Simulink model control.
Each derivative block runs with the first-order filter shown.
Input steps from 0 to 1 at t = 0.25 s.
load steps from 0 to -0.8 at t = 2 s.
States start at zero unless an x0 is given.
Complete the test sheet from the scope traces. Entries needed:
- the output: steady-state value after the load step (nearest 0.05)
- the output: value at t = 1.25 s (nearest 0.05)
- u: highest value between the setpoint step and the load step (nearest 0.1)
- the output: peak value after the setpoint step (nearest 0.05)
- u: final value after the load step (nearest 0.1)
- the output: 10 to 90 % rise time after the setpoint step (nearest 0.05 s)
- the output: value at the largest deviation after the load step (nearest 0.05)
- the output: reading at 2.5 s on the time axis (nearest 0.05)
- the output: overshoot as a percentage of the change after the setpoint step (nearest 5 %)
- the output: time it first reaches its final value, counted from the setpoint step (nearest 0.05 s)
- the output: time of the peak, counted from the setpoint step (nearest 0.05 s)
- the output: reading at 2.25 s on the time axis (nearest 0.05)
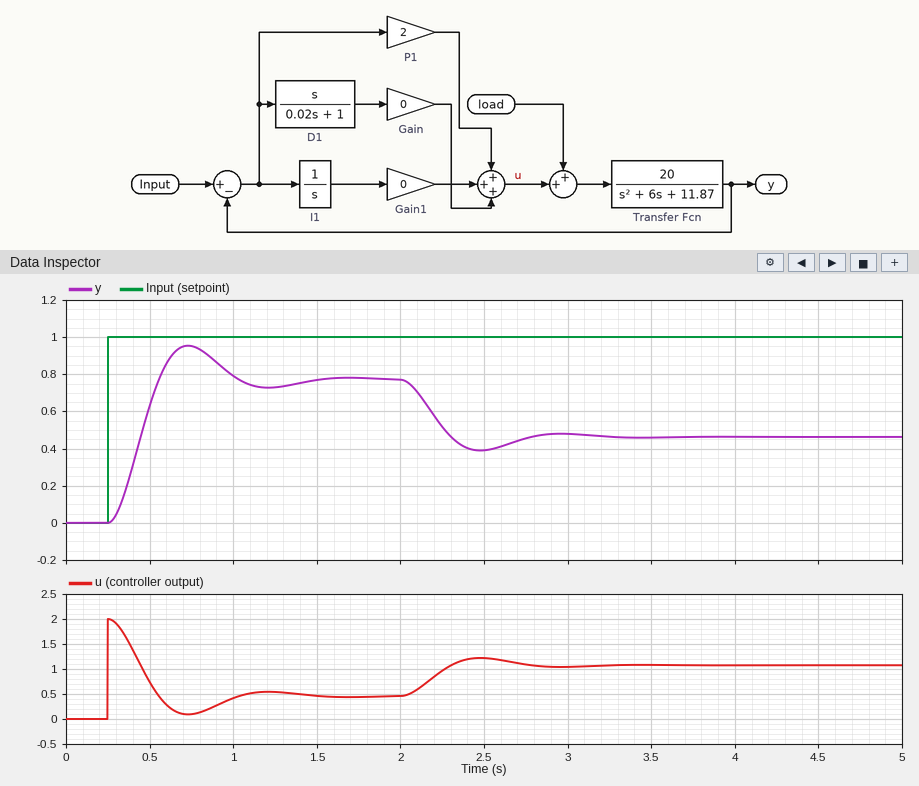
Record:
0.45
0.75
2.0
0.95
1.1
0.20 s
0.40
0.40
25 %
0.30 s
0.50 s
0.50
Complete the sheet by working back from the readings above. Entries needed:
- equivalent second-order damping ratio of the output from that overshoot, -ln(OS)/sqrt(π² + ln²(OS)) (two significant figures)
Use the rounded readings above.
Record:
0.40
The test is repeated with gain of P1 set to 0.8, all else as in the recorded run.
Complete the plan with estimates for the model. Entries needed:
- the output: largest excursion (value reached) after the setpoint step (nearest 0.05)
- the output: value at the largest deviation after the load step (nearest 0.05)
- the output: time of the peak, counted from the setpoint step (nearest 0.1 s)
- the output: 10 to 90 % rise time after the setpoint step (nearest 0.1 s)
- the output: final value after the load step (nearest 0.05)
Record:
0.65
-0.05
0.7 s
0.3 s
0.00
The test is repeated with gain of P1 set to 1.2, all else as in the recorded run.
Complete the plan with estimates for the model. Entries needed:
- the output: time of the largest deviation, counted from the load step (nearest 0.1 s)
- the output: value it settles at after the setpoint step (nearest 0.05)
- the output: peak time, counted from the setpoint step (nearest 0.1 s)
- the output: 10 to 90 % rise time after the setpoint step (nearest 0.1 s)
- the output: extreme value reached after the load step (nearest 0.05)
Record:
0.6 s
0.65
0.6 s
0.3 s
0.15
